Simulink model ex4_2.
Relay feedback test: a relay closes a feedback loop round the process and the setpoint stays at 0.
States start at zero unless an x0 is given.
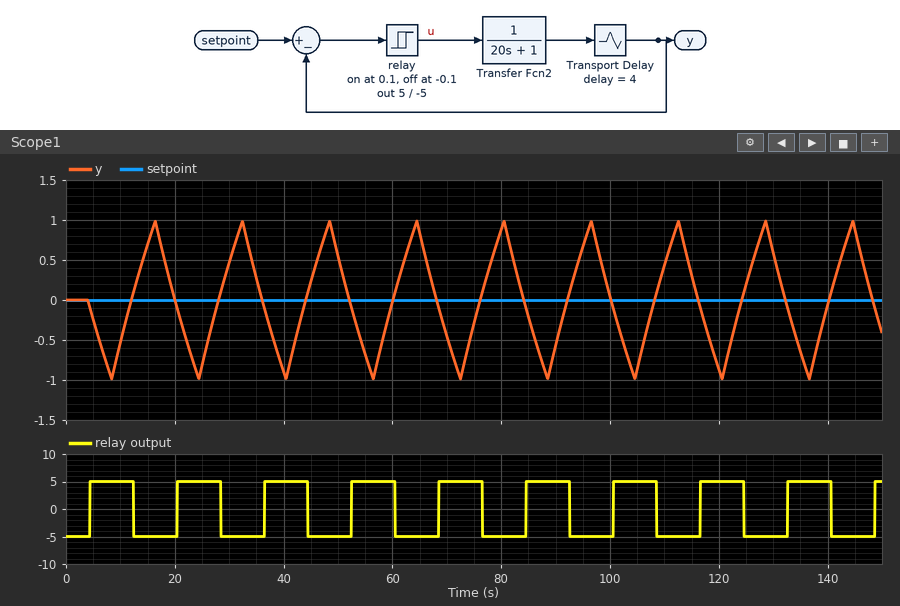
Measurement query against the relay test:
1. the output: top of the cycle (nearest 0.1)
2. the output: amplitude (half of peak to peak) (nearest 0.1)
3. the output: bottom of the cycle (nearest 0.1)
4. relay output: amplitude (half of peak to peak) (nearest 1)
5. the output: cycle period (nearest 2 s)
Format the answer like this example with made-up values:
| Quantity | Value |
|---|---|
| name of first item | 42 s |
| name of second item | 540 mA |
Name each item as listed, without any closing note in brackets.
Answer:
| Quantity | Value |
|---|---|
| the output: top of the cycle | 1.0 |
| the output: amplitude (half of peak to peak) | 1.0 |
| the output: bottom of the cycle | -1.0 |
| relay output: amplitude (half of peak to peak) | 5 |
| the output: cycle period | 16 s |
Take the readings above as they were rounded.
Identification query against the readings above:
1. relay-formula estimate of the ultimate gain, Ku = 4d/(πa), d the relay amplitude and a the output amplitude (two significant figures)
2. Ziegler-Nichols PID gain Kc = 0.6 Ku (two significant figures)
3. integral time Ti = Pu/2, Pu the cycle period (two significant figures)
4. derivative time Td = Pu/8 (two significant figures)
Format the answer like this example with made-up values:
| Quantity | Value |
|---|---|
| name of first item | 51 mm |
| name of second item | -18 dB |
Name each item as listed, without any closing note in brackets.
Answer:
| Quantity | Value |
|---|---|
| relay-formula estimate of the ultimate gain, Ku = 4d/(πa), d the relay amplitude and a the output amplitude | 6.4 |
| Ziegler-Nichols PID gain Kc = 0.6 Ku | 3.8 |
| integral time Ti = Pu/2, Pu the cycle period | 8.0 s |
| derivative time Td = Pu/8 | 2.0 s |
